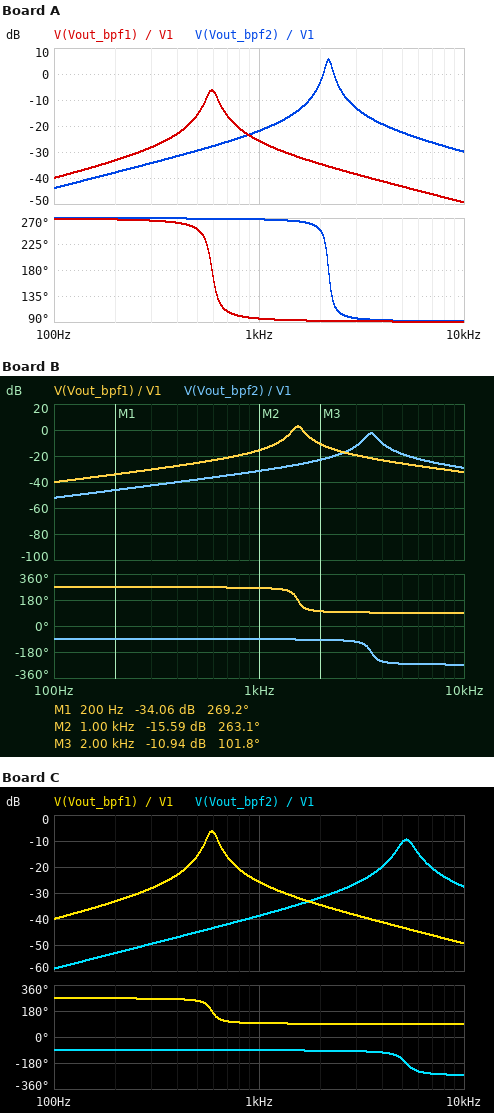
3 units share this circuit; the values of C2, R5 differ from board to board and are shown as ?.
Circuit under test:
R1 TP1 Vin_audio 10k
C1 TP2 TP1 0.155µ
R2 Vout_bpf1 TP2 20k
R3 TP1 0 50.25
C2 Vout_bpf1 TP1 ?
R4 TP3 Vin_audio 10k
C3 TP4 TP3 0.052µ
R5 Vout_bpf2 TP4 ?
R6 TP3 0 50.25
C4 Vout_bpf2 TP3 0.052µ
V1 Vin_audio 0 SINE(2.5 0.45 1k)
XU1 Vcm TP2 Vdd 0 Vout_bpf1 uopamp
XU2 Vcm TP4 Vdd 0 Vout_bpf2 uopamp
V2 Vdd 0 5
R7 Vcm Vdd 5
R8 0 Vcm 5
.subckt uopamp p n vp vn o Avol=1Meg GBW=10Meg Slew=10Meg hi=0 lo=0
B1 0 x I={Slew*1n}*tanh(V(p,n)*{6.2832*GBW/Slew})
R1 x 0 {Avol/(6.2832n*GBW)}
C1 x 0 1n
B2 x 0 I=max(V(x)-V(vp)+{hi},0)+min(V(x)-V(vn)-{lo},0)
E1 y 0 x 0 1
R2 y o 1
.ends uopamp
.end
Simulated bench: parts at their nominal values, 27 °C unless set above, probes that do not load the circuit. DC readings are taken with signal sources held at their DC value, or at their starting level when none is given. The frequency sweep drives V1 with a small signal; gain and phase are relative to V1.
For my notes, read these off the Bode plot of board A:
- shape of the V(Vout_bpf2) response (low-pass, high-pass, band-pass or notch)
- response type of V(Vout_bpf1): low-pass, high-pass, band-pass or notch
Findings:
band-pass
band-pass
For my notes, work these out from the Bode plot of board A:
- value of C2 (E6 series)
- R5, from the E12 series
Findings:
470 nF
39 kΩ
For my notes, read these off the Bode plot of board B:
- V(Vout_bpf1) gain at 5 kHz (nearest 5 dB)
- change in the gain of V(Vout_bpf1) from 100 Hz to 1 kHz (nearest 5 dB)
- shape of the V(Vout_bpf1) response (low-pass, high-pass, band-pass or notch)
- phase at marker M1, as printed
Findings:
-25 dB
25 dB
band-pass
269.2 deg
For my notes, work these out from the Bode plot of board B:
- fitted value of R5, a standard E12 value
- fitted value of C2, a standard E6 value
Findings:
15 kΩ
68 nF
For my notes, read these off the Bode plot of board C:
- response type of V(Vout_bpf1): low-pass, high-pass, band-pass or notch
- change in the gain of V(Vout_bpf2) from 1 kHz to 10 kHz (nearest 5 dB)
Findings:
band-pass
10 dB
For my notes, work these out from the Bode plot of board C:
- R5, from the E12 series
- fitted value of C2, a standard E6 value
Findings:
6.8 kΩ
470 nF
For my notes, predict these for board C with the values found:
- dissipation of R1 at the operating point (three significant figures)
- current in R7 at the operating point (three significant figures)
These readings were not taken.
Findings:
619 µW
500 mA
